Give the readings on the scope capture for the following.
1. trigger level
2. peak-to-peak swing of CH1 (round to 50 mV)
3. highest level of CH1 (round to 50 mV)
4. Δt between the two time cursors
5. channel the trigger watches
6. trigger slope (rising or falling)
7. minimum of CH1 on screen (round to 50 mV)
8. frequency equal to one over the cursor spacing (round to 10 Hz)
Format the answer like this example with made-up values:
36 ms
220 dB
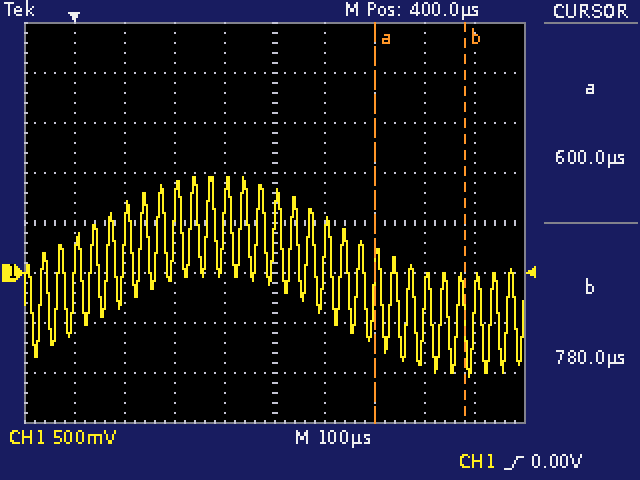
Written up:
0.00 V
2.00 V
950 mV
180 µs
CH1
rising
-1.05 V
5.56 kHz
